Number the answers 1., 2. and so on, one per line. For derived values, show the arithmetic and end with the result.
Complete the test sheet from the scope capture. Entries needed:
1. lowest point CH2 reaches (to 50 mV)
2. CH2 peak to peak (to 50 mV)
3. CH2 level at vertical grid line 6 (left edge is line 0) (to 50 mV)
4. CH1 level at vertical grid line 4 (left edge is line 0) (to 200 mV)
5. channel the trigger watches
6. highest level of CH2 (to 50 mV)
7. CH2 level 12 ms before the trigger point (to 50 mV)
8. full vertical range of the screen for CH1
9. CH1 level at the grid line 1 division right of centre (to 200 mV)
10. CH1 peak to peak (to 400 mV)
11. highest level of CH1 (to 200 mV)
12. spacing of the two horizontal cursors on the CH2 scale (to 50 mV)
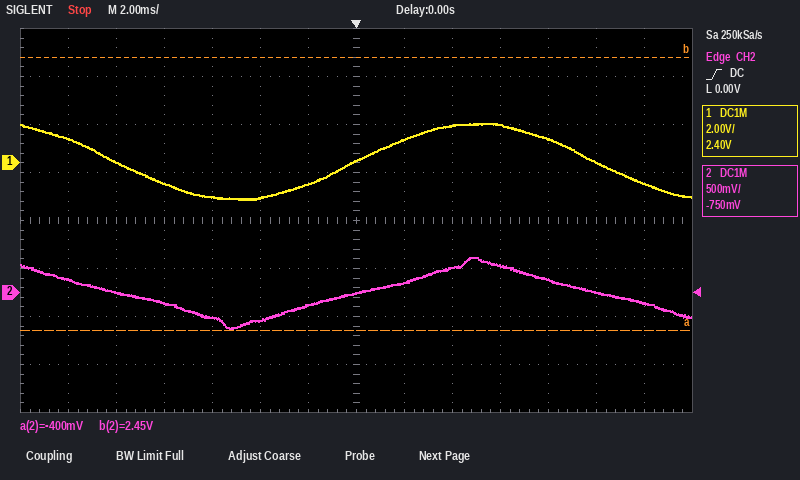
1. -400 mV
2. 350 mV − (-400 mV) = 750 mV
3. -150 mV
4. -1.4 V
5. CH2
6. 350 mV
7. 150 mV
8. 16 V
9. 1.0 V
10. 3.2 V
11. 1.6 V
12. 2.85 V
